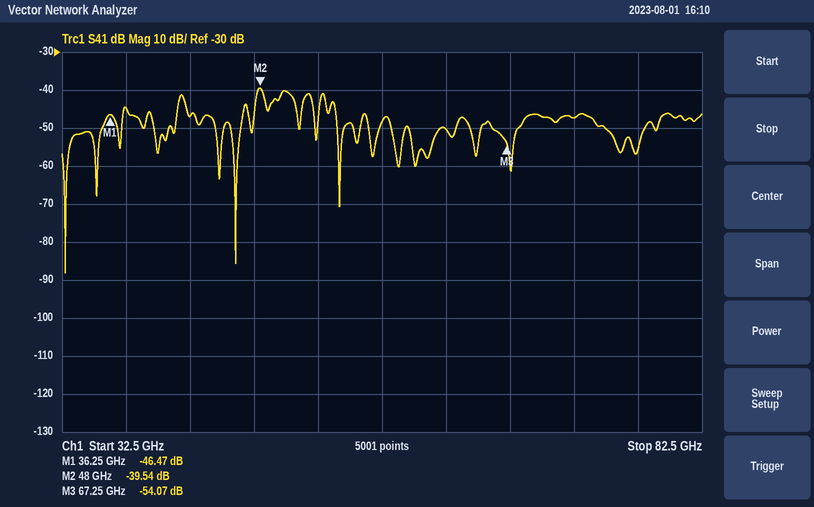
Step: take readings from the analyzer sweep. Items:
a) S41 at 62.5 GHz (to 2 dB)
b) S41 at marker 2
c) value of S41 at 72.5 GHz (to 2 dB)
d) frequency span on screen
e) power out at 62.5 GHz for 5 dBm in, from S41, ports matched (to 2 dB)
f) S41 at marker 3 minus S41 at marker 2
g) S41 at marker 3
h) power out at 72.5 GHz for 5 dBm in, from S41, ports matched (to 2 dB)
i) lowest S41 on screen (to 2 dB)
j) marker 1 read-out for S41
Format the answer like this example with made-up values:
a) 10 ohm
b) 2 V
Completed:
a) -50 dB
b) -39.54 dB
c) -48 dB
d) 50 GHz
e) -46 dBm
f) -14.53 dB
g) -54.07 dB
h) -42 dBm
i) -88 dB
j) -46.47 dB
